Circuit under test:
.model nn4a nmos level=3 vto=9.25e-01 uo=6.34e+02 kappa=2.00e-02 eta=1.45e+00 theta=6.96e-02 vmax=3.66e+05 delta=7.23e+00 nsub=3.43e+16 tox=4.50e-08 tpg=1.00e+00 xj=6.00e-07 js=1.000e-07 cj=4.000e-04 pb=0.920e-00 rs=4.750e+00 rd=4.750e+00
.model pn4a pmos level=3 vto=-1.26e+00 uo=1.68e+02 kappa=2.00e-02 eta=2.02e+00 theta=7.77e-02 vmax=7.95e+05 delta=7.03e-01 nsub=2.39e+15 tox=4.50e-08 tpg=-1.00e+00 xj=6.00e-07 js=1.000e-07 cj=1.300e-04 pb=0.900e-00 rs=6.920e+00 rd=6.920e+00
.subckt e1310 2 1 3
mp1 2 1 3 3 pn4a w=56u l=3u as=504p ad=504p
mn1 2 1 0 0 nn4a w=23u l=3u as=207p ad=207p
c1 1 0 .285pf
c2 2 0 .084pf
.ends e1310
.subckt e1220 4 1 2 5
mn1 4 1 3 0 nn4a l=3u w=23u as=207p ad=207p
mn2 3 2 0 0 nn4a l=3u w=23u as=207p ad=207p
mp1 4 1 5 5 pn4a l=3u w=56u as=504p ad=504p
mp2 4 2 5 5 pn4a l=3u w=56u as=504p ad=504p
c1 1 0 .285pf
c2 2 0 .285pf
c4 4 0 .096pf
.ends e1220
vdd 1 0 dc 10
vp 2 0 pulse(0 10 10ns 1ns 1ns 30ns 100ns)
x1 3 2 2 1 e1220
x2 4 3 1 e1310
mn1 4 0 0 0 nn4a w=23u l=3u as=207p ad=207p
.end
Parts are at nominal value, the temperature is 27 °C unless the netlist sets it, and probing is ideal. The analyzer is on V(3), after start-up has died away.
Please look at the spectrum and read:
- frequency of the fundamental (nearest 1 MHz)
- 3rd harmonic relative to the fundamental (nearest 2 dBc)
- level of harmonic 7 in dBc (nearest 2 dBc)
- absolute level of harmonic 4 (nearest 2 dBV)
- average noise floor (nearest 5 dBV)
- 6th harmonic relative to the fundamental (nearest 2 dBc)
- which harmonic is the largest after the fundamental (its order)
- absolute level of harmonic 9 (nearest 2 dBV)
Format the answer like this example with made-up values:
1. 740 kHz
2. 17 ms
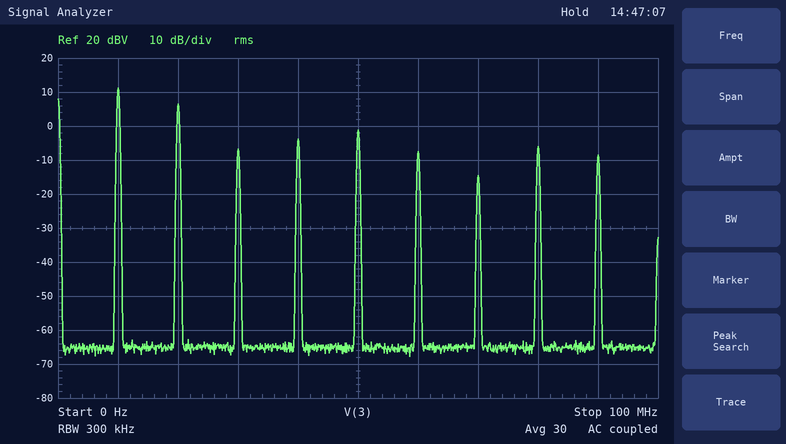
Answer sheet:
1. 10 MHz
2. -18 dBc
3. -26 dBc
4. -4 dBV
5. -65 dBV
6. -18 dBc
7. 2
8. -8 dBV
